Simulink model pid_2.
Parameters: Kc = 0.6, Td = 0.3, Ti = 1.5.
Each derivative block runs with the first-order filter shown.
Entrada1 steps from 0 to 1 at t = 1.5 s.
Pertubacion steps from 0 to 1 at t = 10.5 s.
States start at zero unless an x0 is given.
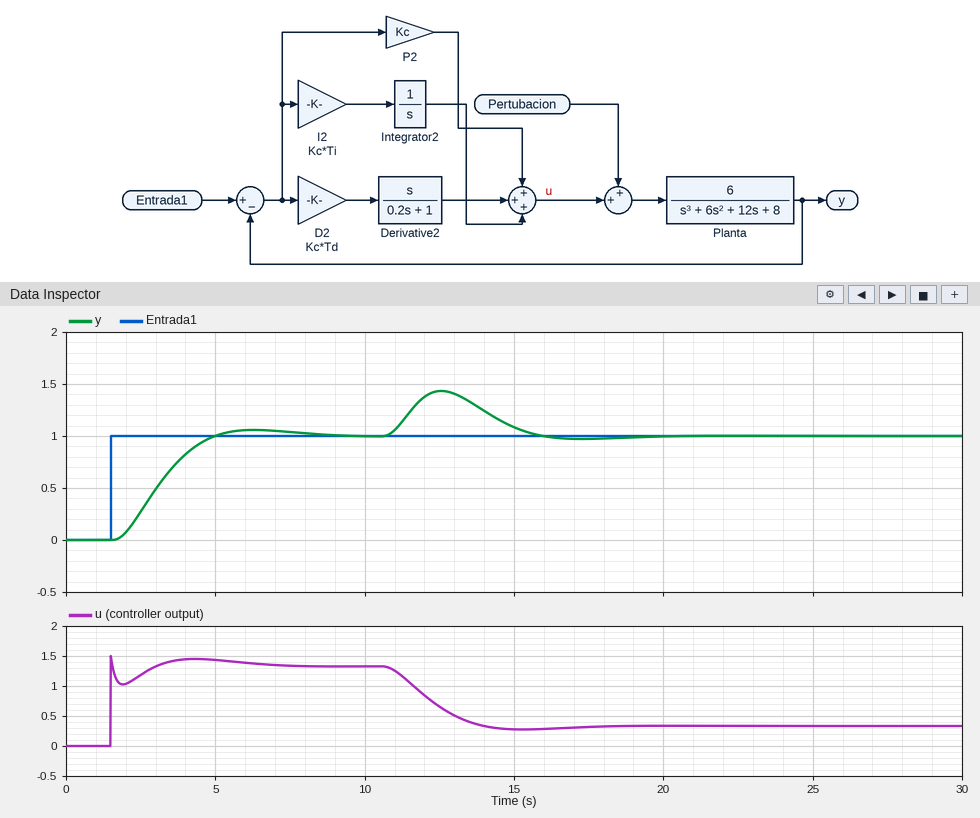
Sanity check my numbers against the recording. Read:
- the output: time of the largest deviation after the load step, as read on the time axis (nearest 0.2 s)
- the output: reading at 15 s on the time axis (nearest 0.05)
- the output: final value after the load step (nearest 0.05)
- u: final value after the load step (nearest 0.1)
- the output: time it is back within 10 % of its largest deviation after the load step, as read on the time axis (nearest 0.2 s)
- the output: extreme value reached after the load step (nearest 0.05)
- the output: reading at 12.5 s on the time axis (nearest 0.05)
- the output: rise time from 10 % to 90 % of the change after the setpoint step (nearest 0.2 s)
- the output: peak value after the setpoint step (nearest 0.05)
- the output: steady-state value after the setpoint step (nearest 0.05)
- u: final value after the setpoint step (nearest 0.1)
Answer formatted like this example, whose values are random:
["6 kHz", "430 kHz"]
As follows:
["12.6 s", "1.10", "1.00", "0.3", "15.4 s", "1.45", "1.45", "2.2 s", "1.05", "1.00", "1.3"]
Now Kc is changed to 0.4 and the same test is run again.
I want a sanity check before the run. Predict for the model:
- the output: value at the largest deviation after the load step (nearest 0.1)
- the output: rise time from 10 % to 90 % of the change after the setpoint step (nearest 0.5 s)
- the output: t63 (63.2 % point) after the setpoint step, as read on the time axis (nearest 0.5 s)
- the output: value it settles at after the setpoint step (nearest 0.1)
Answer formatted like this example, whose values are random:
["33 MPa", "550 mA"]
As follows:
["1.5", "3.5 s", "4.0 s", "1.0"]
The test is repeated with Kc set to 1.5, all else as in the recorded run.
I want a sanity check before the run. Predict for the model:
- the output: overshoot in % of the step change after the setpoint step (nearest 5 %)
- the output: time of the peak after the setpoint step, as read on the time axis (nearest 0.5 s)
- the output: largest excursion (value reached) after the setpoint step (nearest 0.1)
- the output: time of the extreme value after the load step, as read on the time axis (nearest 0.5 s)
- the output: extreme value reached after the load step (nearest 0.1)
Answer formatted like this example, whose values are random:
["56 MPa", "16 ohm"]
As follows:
["20 %", "4.0 s", "1.2", "12.0 s", "1.3"]
